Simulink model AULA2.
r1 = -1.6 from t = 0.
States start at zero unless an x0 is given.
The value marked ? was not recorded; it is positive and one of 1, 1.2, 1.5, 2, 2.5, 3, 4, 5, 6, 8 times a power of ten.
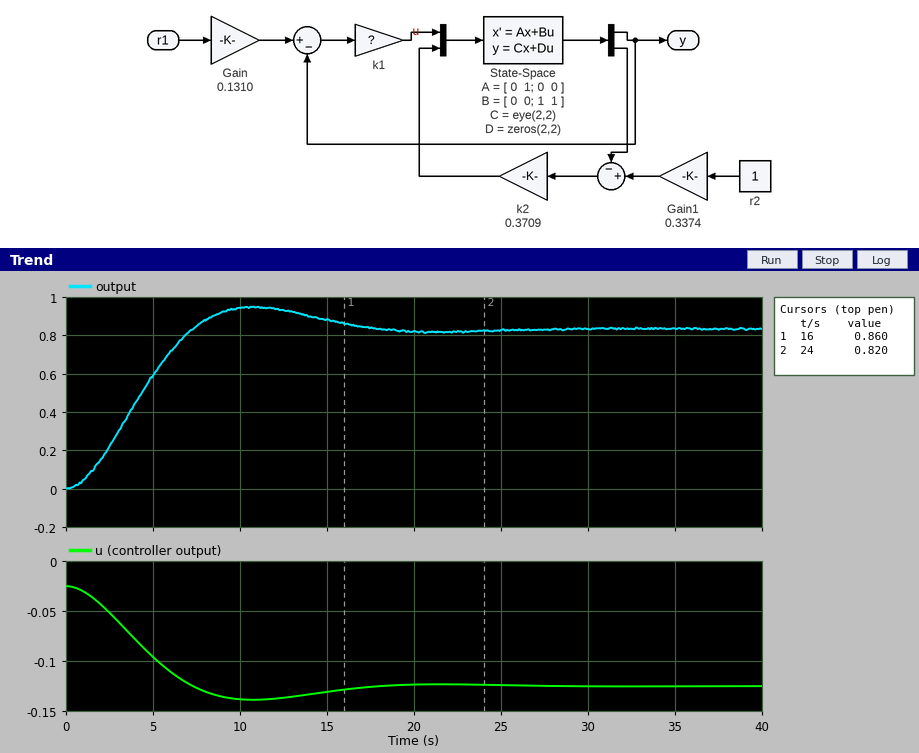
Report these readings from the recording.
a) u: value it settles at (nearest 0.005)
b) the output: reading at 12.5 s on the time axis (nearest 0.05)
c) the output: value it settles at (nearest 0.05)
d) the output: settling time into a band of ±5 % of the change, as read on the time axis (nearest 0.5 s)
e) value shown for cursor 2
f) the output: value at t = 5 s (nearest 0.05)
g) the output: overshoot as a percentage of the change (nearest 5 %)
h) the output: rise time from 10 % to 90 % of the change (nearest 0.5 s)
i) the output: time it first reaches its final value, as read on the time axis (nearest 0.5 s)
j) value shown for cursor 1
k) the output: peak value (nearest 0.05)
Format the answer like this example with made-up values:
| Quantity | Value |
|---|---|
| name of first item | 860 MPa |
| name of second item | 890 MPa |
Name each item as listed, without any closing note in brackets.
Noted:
| Quantity | Value |
|---|---|
| u: value it settles at | -0.125 |
| the output: reading at 12.5 s on the time axis | 0.95 |
| the output: value it settles at | 0.85 |
| the output: settling time into a band of ±5 % of the change, as read on the time axis | 15.5 s |
| value shown for cursor 2 | 0.820 |
| the output: value at t = 5 s | 0.60 |
| the output: overshoot as a percentage of the change | 15 % |
| the output: rise time from 10 % to 90 % of the change | 5.0 s |
| the output: time it first reaches its final value, as read on the time axis | 7.5 s |
| value shown for cursor 1 | 0.860 |
| the output: peak value | 0.95 |
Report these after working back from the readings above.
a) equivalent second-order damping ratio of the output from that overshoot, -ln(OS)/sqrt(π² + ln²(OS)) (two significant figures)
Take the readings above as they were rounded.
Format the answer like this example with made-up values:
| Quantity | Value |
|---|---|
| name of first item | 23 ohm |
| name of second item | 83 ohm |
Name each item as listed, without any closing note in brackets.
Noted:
| Quantity | Value |
|---|---|
| equivalent second-order damping ratio of the output from that overshoot, -ln(OS)/sqrt(π² + ln²(OS)) | 0.52 |
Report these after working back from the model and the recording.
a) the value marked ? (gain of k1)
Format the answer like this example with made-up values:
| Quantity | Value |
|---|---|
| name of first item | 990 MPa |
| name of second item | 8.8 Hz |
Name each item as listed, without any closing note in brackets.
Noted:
| Quantity | Value |
|---|---|
| the value marked ? | 0.12 |
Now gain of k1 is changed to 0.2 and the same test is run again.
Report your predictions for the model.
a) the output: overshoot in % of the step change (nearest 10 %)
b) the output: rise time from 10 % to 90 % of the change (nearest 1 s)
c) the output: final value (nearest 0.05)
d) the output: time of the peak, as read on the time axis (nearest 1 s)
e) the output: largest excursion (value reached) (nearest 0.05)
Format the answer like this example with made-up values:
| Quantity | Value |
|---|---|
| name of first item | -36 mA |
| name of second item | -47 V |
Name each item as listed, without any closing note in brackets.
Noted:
| Quantity | Value |
|---|---|
| the output: overshoot in % of the step change | 20 % |
| the output: rise time from 10 % to 90 % of the change | 3 s |
| the output: final value | 0.40 |
| the output: time of the peak, as read on the time axis | 8 s |
| the output: largest excursion (value reached) | 0.50 |
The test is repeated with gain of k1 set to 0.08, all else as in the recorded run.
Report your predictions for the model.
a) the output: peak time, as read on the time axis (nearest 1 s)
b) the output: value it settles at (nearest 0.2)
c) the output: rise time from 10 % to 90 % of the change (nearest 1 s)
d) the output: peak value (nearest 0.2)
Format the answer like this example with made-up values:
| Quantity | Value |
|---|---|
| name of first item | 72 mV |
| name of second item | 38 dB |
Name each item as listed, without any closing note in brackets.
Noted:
| Quantity | Value |
|---|---|
| the output: peak time, as read on the time axis | 15 s |
| the output: value it settles at | 1.4 |
| the output: rise time from 10 % to 90 % of the change | 7 s |
| the output: peak value | 1.4 |
